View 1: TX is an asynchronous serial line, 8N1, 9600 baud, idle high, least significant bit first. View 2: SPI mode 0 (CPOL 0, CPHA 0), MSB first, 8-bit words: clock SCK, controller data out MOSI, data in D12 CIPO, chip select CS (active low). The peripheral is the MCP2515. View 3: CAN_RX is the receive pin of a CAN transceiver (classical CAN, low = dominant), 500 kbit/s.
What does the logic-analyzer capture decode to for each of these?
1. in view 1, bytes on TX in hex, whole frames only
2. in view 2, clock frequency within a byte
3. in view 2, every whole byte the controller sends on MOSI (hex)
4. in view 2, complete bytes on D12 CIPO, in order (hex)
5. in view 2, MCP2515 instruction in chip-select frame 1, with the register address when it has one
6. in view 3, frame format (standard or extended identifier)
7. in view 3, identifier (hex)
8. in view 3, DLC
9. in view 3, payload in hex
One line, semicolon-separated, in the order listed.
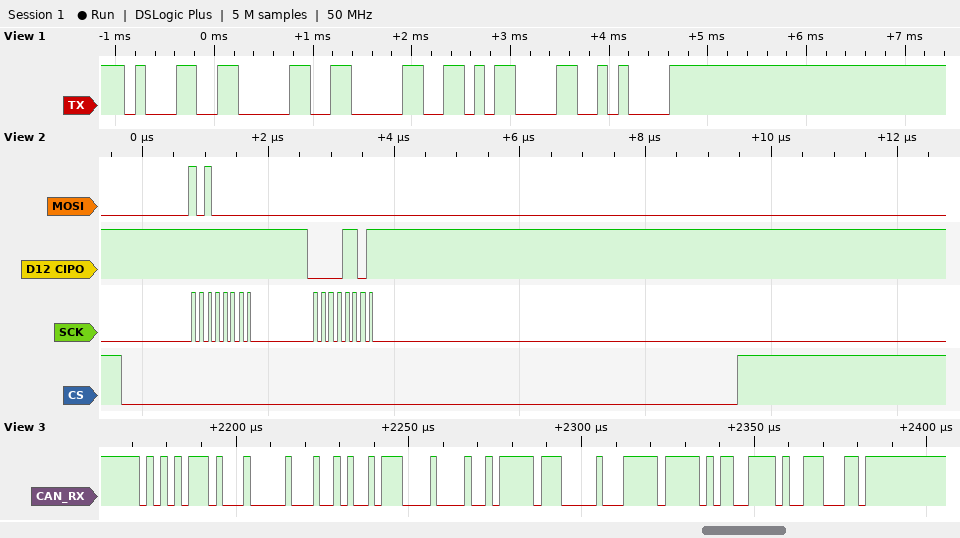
0x31 0x30 0x30 0x0D 0x0A; 8 MHz; 0xA0 0x00; 0xFF 0x0D; READ STATUS; standard; 0x55D; 8; 04 A5 C2 12 FF 00 FF EC
